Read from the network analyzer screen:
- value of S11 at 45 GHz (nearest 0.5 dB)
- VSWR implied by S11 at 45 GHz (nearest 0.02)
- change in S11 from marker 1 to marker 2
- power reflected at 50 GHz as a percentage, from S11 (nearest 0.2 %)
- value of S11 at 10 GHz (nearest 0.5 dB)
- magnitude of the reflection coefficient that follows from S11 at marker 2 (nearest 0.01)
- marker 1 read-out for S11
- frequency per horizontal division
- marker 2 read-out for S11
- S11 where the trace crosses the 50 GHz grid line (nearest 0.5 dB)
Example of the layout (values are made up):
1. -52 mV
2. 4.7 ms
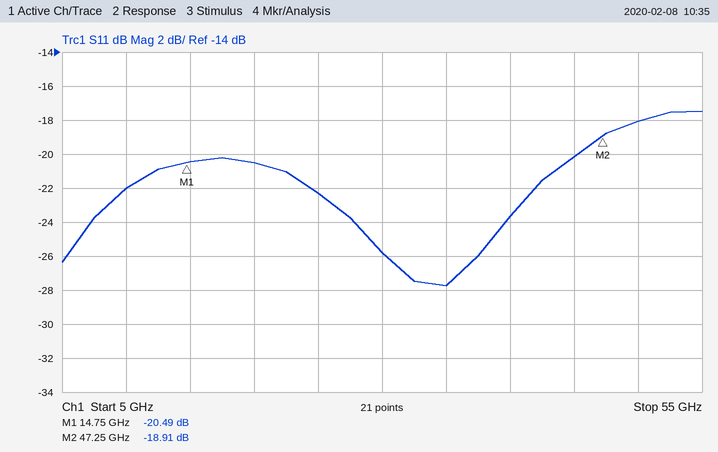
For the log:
1. -20.0 dB
2. 1.22
3. 1.58 dB
4. 1.6 %
5. -22.0 dB
6. 0.11
7. -20.49 dB
8. 5 GHz
9. -18.91 dB
10. -18.0 dB
